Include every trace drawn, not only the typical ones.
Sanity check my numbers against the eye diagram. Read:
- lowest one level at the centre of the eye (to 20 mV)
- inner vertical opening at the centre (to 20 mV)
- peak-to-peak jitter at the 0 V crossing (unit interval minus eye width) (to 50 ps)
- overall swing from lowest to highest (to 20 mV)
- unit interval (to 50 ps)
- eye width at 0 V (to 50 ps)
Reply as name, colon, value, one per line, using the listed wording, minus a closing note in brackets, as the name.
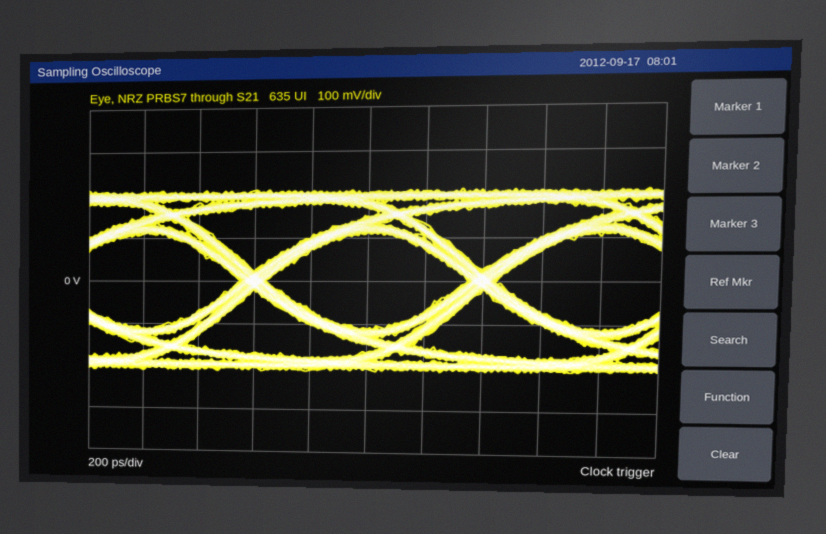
lowest one level at the centre of the eye: 120 mV
inner vertical opening at the centre: 220 mV
peak-to-peak jitter at the 0 V crossing (unit interval minus eye width): 100 ps
overall swing from lowest to highest: 420 mV
unit interval: 800 ps
eye width at 0 V: 700 ps
